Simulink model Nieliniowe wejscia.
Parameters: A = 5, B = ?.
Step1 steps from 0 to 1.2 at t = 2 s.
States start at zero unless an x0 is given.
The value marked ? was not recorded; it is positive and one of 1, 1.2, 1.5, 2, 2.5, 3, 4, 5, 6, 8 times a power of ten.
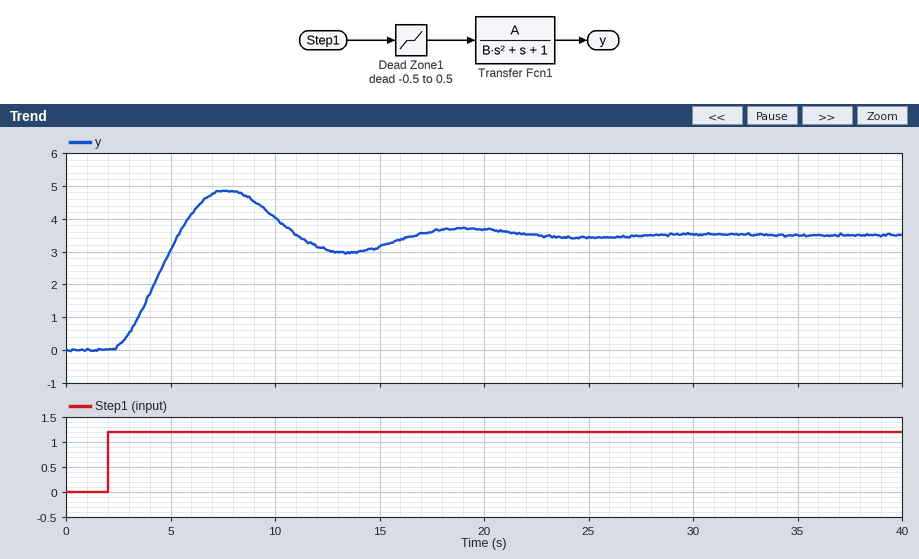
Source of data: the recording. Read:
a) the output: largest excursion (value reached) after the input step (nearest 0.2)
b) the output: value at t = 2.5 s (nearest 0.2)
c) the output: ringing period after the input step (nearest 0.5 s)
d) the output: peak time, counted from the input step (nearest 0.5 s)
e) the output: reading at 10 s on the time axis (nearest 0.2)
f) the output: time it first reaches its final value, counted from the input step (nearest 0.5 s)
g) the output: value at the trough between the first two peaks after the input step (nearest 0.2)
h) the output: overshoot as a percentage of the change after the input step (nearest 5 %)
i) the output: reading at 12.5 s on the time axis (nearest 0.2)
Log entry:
4.8
0.2
11.5 s
5.5 s
4.0
3.5 s
3.0
40 %
3.0
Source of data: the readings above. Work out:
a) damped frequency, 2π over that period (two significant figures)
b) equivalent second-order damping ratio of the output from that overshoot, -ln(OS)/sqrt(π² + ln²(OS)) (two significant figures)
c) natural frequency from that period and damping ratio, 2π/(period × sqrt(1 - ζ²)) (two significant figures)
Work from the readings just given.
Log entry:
0.55 rad/s
0.28
0.57 rad/s
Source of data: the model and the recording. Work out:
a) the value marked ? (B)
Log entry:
3
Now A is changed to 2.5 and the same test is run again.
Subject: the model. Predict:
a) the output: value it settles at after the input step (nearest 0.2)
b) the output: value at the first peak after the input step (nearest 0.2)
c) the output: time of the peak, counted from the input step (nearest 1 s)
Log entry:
1.8
2.4
6 s
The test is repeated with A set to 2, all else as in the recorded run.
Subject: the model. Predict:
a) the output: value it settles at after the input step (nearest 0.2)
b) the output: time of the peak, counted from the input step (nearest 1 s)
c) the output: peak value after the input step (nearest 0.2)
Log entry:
1.4
6 s
2.0
